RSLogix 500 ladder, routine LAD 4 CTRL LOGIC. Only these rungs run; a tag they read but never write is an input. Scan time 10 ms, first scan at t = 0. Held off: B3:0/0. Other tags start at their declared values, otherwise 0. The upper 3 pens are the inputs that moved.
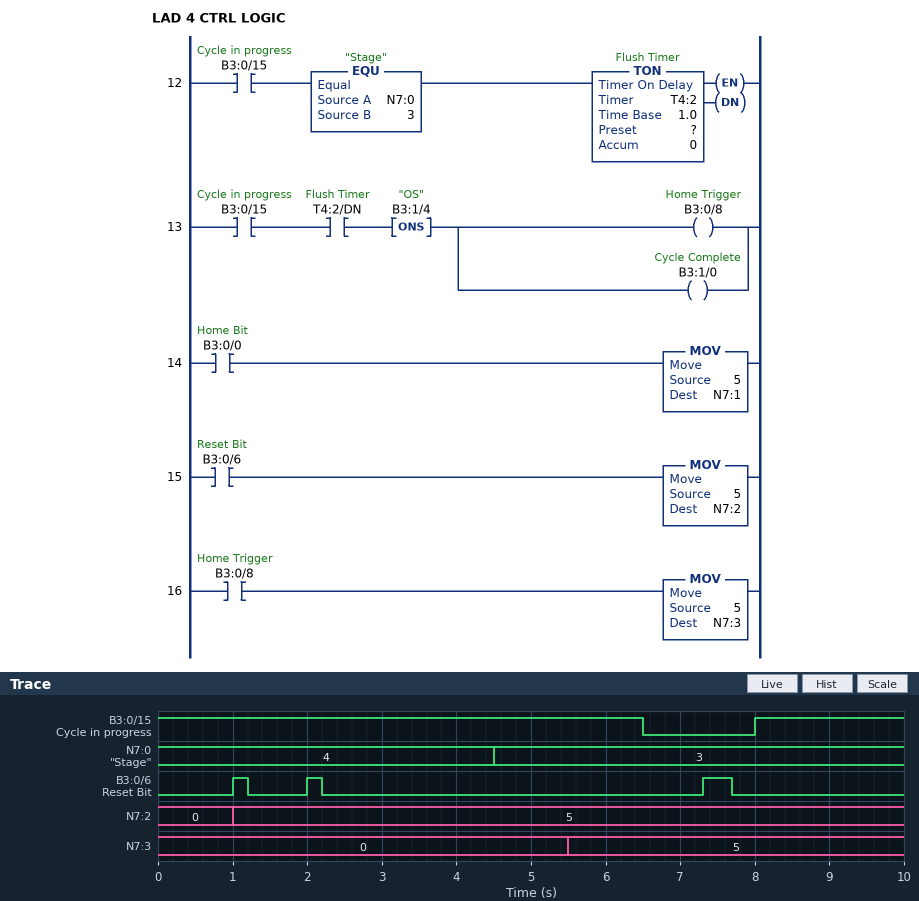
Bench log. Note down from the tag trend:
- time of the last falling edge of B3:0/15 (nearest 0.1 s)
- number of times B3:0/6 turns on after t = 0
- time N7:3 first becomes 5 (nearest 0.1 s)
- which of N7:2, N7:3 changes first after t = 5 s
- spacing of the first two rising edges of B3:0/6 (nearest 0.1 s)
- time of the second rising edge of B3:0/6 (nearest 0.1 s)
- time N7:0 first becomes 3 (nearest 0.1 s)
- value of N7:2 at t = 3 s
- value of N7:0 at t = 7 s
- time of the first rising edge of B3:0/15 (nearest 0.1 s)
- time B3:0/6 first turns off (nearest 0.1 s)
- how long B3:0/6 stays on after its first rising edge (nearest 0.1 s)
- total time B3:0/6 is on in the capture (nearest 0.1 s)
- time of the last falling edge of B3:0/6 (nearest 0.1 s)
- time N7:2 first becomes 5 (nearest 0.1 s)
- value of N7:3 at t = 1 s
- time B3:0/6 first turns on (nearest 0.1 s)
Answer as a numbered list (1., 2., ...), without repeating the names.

1. 6.5 s
2. 3
3. 5.5 s
4. N7:3
5. 1.0 s
6. 2.0 s
7. 4.5 s
8. 5
9. 3
10. 8.0 s
11. 1.2 s
12. 0.2 s
13. 0.8 s
14. 7.7 s
15. 1.0 s
16. 0
17. 1.0 s
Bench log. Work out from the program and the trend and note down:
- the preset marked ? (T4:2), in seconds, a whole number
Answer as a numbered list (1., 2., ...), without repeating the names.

1. 1 s
